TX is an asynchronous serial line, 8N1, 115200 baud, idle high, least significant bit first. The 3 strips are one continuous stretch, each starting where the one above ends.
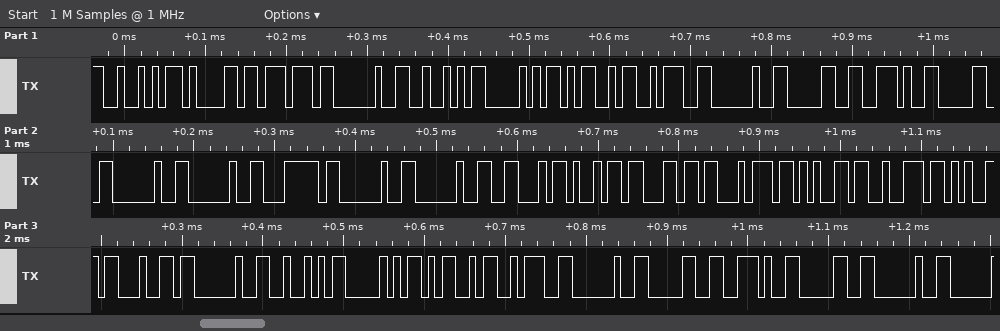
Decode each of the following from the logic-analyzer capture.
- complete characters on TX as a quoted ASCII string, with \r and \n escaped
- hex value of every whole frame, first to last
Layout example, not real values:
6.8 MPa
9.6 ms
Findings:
"Raw RPM: 0.0  |  Filtered RPM: 0.0 "
52 61 77 20 52 50 4D 3A 20 30 2E 30 20 20 7C 20 20 46 69 6C 74 65 72 65 64 20 52 50 4D 3A 20 30 2E 30 20
